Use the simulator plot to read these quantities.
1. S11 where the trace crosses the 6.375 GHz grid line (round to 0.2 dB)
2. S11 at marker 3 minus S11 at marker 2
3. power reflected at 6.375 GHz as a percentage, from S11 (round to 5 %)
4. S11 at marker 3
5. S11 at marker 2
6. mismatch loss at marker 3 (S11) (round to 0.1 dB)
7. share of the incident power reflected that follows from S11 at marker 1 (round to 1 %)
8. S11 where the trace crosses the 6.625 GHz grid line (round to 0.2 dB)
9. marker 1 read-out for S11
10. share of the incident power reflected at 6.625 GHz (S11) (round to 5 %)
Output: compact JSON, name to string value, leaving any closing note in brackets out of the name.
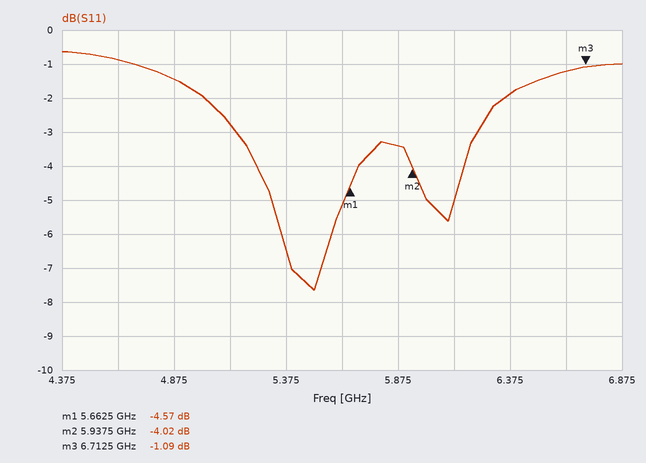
{"S11 where the trace crosses the 6.375 GHz grid line": "-1.8 dB", "S11 at marker 3 minus S11 at marker 2": "2.93 dB", "power reflected at 6.375 GHz as a percentage, from S11": "65 %", "S11 at marker 3": "-1.09 dB", "S11 at marker 2": "-4.02 dB", "mismatch loss at marker 3 (S11)": "6.5 dB", "share of the incident power reflected that follows from S11 at marker 1": "35 %", "S11 where the trace crosses the 6.625 GHz grid line": "-1.2 dB", "marker 1 read-out for S11": "-4.57 dB", "share of the incident power reflected at 6.625 GHz (S11)": "75 %"}
